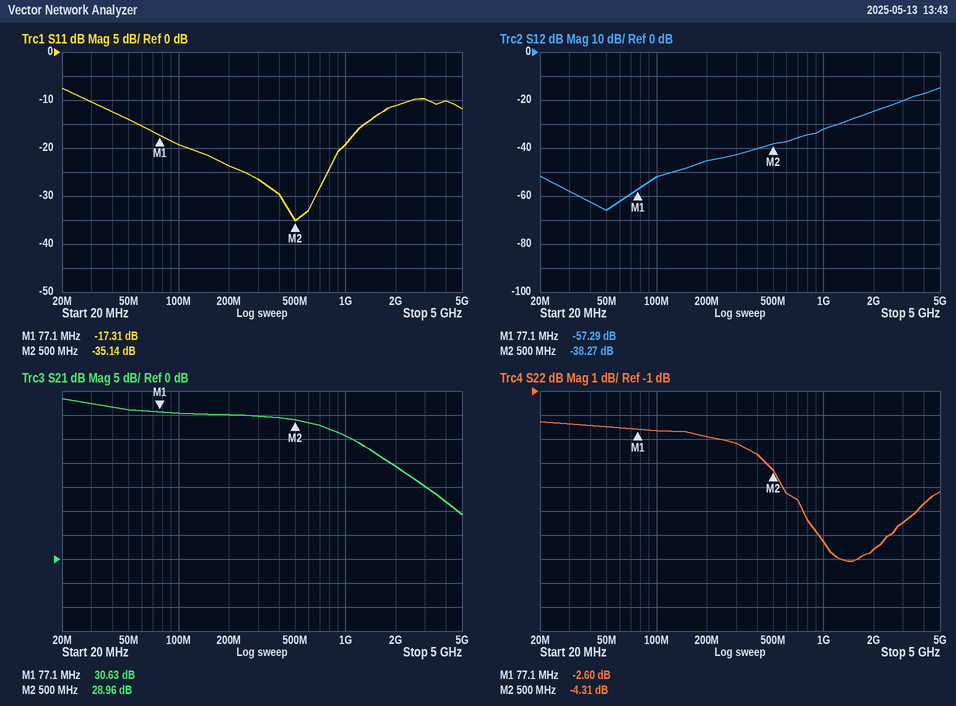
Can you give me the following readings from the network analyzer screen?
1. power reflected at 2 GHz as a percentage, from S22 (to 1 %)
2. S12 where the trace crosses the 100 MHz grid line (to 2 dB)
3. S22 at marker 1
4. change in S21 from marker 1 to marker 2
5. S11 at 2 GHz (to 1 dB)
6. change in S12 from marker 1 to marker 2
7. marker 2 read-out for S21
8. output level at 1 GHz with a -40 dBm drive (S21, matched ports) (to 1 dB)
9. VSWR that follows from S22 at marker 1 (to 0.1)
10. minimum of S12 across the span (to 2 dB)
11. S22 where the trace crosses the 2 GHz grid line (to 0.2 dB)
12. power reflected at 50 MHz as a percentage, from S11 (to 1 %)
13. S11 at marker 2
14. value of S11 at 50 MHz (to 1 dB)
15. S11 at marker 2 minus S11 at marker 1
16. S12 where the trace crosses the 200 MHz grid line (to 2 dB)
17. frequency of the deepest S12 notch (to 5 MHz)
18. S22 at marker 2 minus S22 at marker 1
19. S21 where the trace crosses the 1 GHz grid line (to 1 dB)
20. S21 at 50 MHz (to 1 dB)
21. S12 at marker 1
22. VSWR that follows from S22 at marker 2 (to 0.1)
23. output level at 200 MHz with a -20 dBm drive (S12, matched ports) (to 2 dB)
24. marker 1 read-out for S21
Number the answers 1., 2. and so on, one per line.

1. 17 %
2. -52 dB
3. -2.60 dB
4. -1.67 dB
5. -11 dB
6. 19.02 dB
7. 28.96 dB
8. -14 dBm
9. 6.7
10. -66 dB
11. -7.6 dB
12. 4 %
13. -35.14 dB
14. -14 dB
15. -17.83 dB
16. -46 dB
17. 50 MHz
18. -1.71 dB
19. 26 dB
20. 31 dB
21. -57.29 dB
22. 4.1
23. -66 dBm
24. 30.63 dB
